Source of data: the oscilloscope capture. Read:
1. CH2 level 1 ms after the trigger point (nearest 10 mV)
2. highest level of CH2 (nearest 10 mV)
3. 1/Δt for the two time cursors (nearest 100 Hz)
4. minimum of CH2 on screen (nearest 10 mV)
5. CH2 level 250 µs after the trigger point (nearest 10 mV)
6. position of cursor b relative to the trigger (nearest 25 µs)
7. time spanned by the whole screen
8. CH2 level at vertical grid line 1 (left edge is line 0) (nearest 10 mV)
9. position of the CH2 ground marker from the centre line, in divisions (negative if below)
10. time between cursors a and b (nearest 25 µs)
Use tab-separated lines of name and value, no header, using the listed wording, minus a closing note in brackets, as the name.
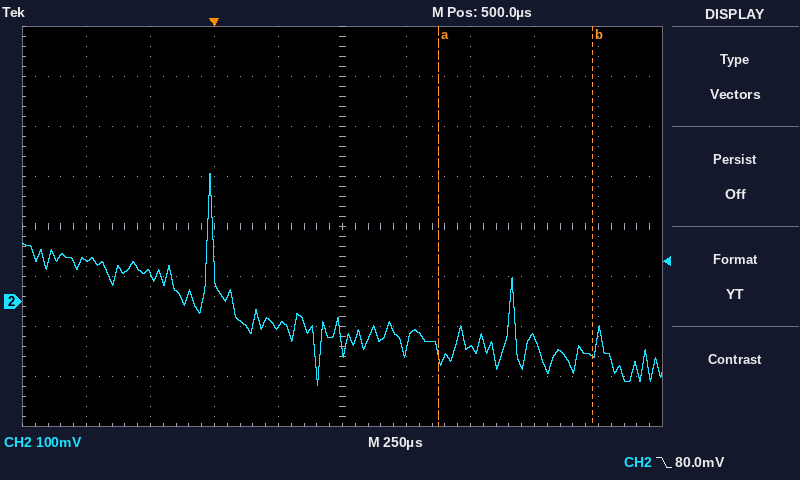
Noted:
CH2 level 1 ms after the trigger point	-90 mV
highest level of CH2	260 mV
1/Δt for the two time cursors	1.7 kHz
minimum of CH2 on screen	-170 mV
CH2 level 250 µs after the trigger point	-50 mV
position of cursor b relative to the trigger	+1.475 ms
time spanned by the whole screen	2.5 ms
CH2 level at vertical grid line 1 (left edge is line 0)	80 mV
position of the CH2 ground marker from the centre line, in divisions	-1.5 div
time between cursors a and b	600 µs
